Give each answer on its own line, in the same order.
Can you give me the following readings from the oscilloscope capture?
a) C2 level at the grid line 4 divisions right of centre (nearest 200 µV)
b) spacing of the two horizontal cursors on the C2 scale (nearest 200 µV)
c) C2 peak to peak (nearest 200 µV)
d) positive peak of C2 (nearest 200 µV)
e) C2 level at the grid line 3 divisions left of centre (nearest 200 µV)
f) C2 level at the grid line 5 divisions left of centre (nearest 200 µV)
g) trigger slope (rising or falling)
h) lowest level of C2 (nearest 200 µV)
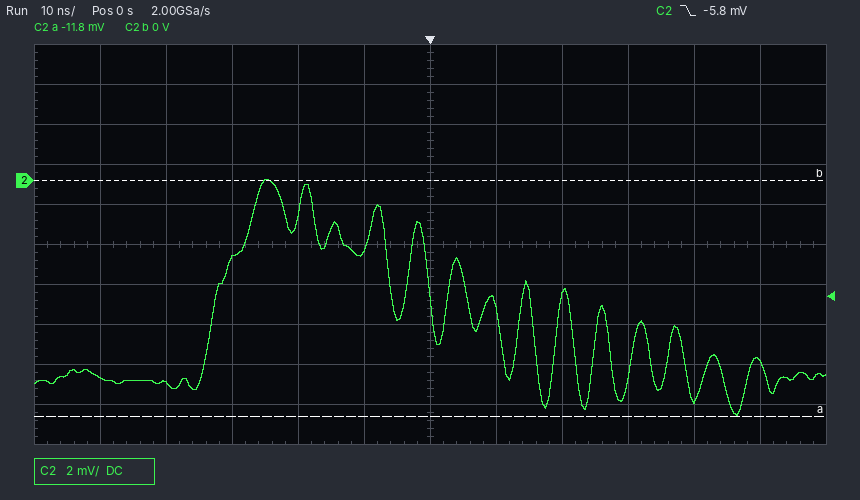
-11.0 mV
11.8 mV
11.8 mV
0.0 mV
-4.0 mV
-9.8 mV
falling
-11.8 mV
